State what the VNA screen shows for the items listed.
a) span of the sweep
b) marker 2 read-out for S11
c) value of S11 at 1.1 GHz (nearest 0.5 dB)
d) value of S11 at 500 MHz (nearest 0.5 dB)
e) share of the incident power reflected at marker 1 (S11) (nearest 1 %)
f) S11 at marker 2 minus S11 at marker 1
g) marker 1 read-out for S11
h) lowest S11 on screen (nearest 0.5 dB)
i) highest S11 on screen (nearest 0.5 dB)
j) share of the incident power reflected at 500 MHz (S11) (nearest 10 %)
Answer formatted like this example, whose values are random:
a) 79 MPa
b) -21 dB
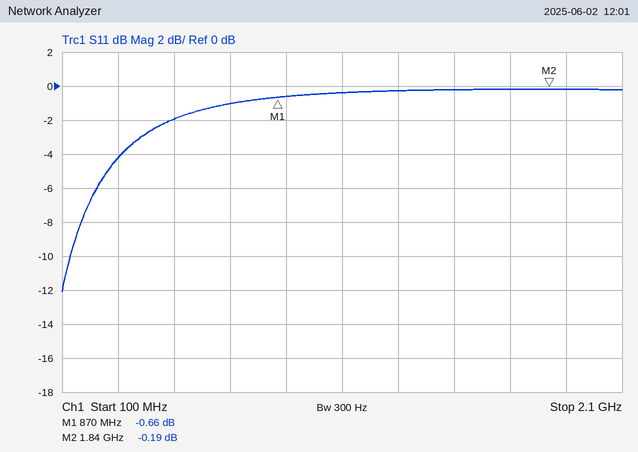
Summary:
a) 2 GHz
b) -0.19 dB
c) -0.5 dB
d) -2.0 dB
e) 86 %
f) 0.47 dB
g) -0.66 dB
h) -12.0 dB
i) 0.0 dB
j) 60 %
